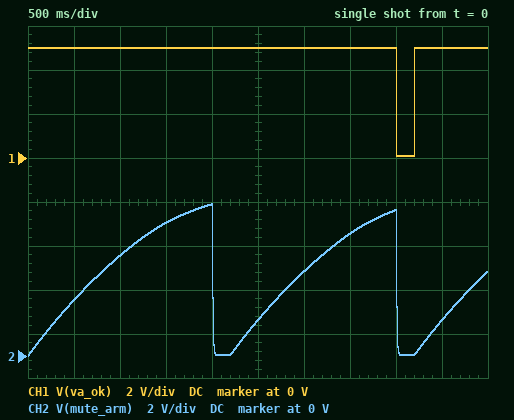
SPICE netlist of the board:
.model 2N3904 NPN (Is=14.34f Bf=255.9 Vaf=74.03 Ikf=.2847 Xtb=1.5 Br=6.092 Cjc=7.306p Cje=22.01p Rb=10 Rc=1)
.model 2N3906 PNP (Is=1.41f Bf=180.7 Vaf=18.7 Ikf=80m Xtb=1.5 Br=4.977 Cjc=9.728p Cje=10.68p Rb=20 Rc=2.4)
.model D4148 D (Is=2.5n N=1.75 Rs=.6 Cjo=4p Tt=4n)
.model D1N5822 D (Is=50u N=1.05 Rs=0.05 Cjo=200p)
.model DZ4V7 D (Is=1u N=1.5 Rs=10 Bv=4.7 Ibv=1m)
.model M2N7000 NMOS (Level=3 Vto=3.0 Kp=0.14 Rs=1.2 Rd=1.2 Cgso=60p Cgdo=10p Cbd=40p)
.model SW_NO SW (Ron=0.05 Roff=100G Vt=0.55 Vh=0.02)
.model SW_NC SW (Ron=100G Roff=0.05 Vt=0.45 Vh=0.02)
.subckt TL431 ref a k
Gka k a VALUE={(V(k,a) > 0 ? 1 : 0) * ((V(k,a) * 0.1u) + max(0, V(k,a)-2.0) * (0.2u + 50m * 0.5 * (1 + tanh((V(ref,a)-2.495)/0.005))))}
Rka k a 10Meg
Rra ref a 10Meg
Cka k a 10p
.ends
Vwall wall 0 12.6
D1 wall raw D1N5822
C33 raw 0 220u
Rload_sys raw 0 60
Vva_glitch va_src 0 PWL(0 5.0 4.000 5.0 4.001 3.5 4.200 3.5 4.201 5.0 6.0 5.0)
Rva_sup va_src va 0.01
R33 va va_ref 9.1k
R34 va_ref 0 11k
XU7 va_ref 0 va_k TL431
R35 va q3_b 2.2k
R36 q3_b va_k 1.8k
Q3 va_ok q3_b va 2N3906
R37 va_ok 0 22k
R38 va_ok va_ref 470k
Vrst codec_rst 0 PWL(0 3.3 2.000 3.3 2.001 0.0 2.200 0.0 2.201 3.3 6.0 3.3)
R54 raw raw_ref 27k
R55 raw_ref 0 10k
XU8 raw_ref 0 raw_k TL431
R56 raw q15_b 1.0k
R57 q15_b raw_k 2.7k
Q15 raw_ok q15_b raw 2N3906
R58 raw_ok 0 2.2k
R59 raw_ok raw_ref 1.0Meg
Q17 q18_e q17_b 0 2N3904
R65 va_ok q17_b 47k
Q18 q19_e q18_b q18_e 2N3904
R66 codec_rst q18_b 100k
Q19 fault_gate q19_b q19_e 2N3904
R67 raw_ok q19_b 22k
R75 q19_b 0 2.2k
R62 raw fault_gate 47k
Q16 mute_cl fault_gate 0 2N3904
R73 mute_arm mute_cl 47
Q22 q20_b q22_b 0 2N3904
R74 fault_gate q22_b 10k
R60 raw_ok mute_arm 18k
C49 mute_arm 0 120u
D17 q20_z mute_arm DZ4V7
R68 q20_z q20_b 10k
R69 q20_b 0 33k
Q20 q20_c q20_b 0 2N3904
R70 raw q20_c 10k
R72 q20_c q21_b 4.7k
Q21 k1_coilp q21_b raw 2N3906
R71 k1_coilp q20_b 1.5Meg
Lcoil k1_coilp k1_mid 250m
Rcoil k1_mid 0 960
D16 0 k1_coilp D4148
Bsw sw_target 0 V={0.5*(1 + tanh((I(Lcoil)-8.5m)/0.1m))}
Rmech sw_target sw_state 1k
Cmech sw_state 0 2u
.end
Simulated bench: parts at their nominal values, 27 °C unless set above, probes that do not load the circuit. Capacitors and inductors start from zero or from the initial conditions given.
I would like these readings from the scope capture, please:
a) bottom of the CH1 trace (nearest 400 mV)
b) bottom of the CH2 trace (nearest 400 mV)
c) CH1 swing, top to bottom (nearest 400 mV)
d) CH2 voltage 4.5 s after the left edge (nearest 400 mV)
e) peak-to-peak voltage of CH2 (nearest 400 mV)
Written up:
0 V
0 V
4.8 V
1.6 V
6.8 V
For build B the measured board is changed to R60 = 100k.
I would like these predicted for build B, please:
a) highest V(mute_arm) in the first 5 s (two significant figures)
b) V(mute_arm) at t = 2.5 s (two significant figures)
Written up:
1.9 V
310 mV
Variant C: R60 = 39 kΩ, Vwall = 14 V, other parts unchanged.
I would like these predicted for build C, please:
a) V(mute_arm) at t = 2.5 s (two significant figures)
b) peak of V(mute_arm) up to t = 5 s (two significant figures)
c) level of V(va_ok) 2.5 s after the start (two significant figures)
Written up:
870 mV
4.8 V
5.0 V
